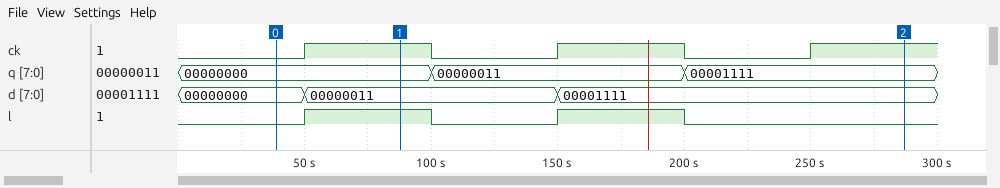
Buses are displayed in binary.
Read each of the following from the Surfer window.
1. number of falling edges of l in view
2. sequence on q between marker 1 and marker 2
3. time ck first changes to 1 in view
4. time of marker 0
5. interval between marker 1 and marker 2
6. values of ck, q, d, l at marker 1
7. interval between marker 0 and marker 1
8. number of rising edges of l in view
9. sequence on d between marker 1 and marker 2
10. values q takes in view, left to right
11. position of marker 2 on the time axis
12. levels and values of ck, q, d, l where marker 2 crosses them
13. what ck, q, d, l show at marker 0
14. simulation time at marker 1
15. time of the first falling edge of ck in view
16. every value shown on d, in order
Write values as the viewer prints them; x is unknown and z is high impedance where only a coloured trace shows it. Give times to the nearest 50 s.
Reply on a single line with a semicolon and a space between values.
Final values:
2; 00000000, 00000011, 00001111; 50 s; 50 s; 200 s; ck=1, q=00000000, d=00000011, l=1; 50 s; 2; 00000011, 00001111; 00000000, 00000011, 00001111; 300 s; ck=1, q=00001111, d=00001111, l=0; ck=0, q=00000000, d=00000000, l=0; 100 s; 100 s; 00000000, 00000011, 00001111
